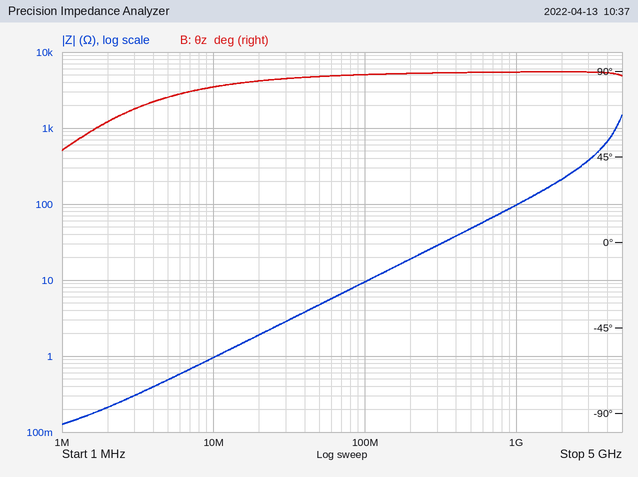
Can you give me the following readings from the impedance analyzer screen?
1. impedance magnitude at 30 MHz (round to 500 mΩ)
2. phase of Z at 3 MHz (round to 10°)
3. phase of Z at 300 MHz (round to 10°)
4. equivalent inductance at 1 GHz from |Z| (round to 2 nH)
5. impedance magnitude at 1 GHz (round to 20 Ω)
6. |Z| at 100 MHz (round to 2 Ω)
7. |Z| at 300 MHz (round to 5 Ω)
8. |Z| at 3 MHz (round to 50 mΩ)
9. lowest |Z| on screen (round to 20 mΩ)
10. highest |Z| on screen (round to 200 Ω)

3.0 Ω
70°
90°
16 nH
100 Ω
10 Ω
30 Ω
300 mΩ
120 mΩ
1.4 kΩ
